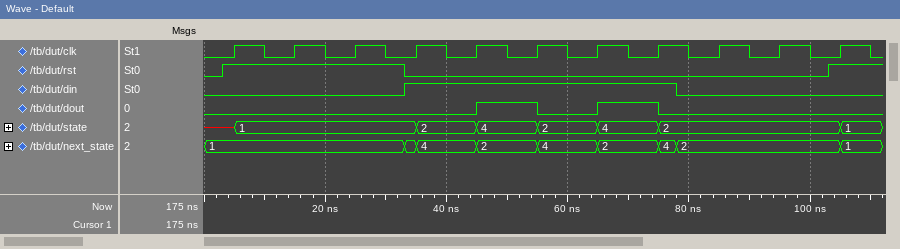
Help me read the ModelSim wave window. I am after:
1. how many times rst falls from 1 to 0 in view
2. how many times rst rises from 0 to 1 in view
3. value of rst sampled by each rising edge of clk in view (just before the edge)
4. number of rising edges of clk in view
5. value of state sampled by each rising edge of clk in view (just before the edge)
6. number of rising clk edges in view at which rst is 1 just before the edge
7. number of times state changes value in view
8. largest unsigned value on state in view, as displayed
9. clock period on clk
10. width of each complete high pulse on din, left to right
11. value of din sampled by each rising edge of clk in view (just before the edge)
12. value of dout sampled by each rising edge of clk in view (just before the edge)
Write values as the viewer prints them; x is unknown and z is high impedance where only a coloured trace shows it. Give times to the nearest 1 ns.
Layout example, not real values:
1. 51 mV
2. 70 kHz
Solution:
1. 1
2. 2
3. 1 1 1 0 0 0 0 0 0 0 1
4. 11
5. x, 1, 1, 1, 2, 4, 2, 4, 2, 2, 2
6. 4
7. 7
8. 4
9. 10 ns
10. 45 ns
11. 0 0 0 1 1 1 1 1 0 0 0
12. 0 0 0 0 0 1 0 1 0 0 0
